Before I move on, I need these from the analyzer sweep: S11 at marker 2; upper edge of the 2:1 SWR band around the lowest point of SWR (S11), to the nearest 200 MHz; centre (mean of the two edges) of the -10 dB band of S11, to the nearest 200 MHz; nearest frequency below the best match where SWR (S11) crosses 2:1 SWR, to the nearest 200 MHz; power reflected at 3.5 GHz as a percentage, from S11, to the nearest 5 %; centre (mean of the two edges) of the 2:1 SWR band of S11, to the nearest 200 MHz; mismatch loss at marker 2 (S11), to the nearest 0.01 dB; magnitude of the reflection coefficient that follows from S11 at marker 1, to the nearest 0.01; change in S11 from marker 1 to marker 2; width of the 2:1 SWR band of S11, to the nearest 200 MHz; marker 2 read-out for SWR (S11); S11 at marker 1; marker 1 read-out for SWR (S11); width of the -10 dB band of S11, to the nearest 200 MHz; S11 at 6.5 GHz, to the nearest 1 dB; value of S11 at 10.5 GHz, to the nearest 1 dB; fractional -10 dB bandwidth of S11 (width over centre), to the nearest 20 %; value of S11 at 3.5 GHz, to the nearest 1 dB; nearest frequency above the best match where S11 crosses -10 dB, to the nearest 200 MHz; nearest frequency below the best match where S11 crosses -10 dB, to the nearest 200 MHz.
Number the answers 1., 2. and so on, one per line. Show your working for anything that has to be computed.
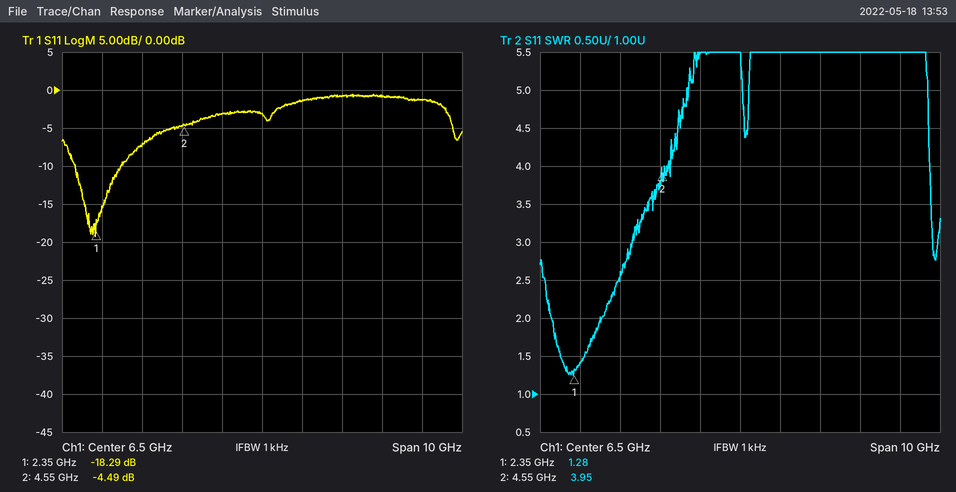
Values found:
1. -4.49 dB
2. 3.0 GHz
3. 2.4 GHz
4. 1.8 GHz
5. 10^(-7/10) ≈ 20 %
6. 2.4 GHz
7. −10 log10(1 − 10^(-4.49/10)) ≈ 1.91 dB
8. 10^(-18.29/20) ≈ 0.12
9. -4.49 − (-18.29) = 13.80 dB
10. 3.0 GHz − 1.8 GHz = 1.2 GHz
11. 3.95
12. -18.29 dB
13. 1.28
14. 3.0 GHz − 1.8 GHz = 1.2 GHz
15. -3 dB
16. -1 dB
17. 1.2 GHz / 2.4 GHz ≈ 50.0 %, so 40 % to the nearest 20 %
18. -7 dB
19. 3.0 GHz
20. 1.8 GHz
